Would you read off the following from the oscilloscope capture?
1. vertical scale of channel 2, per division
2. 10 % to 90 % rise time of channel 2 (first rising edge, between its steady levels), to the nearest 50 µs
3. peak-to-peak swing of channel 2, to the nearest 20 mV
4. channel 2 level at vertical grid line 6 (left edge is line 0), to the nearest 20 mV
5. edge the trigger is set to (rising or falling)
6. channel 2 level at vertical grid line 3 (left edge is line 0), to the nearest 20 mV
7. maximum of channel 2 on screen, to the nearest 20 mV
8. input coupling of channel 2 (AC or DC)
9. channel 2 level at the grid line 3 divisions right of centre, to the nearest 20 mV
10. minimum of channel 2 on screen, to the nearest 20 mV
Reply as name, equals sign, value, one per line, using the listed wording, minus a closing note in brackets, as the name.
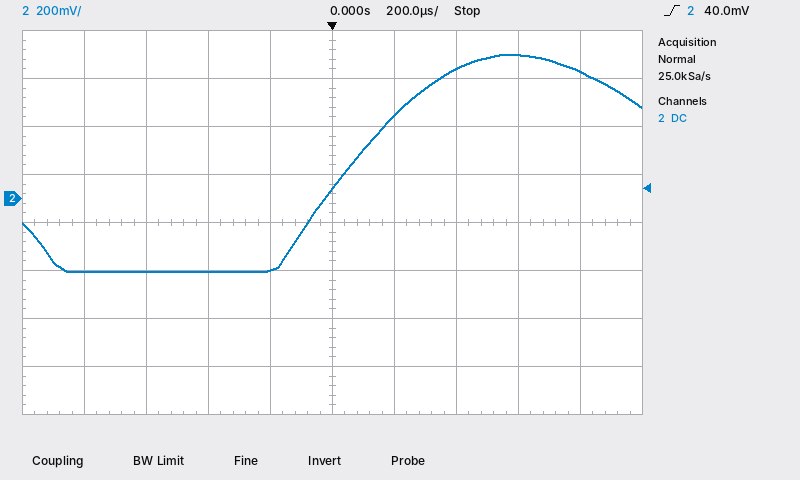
vertical scale of channel 2, per division = 200 mV
10 % to 90 % rise time of channel 2 (first rising edge, between its steady levels), to the nearest 50 µs = 500 µs
peak-to-peak swing of channel 2, to the nearest 20 mV = 900 mV
channel 2 level at vertical grid line 6 (left edge is line 0), to the nearest 20 mV = 340 mV
edge the trigger is set to = rising
channel 2 level at vertical grid line 3 (left edge is line 0), to the nearest 20 mV = -300 mV
maximum of channel 2 on screen, to the nearest 20 mV = 600 mV
input coupling of channel 2 = DC
channel 2 level at the grid line 3 divisions right of centre, to the nearest 20 mV = 600 mV
minimum of channel 2 on screen, to the nearest 20 mV = -300 mV
